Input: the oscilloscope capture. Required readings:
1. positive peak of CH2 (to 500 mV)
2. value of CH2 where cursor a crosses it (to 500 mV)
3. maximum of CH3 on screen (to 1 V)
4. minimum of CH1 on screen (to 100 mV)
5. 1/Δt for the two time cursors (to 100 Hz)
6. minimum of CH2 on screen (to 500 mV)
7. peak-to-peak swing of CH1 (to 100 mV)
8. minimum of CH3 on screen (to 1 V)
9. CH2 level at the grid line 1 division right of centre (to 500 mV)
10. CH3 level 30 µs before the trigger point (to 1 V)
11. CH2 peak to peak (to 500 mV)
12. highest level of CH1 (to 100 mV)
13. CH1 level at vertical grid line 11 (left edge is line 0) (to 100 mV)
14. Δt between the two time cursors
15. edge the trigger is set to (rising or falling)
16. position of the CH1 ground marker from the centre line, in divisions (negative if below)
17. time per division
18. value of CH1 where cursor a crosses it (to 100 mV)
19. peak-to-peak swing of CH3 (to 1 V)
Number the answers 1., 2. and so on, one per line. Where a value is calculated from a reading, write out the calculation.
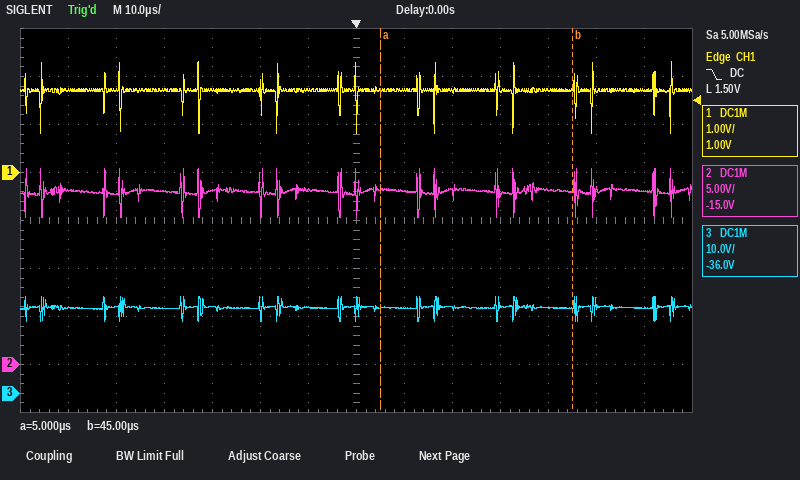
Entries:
1. 20.5 V
2. 18.0 V
3. 20 V
4. 800 mV
5. 1 / 40 µs ≈ 25.0 kHz
6. 15.5 V
7. 2.3 V − (800 mV) = 1.5 V
8. 15 V
9. 18.0 V
10. 18 V
11. 20.5 V − (15.5 V) = 5.0 V
12. 2.3 V
13. 1.7 V
14. 45 µs − (5 µs) = 40 µs
15. falling
16. +1.0 div
17. 10 µs
18. 1.7 V
19. 20 V − (15 V) = 5 V
